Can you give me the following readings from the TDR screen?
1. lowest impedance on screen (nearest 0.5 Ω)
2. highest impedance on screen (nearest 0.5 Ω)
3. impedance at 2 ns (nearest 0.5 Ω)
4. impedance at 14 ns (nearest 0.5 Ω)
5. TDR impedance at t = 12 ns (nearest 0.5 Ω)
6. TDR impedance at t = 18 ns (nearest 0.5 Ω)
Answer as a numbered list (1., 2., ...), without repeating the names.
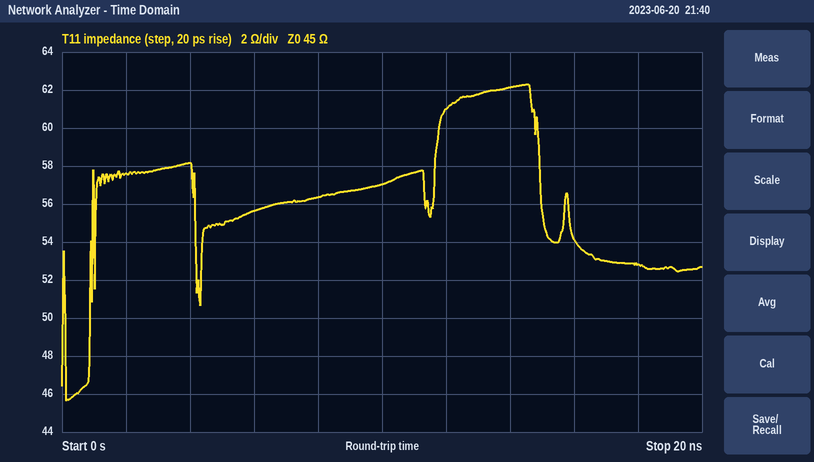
1. 45.5 Ω
2. 62.5 Ω
3. 57.5 Ω
4. 62.0 Ω
5. 61.0 Ω
6. 53.0 Ω
